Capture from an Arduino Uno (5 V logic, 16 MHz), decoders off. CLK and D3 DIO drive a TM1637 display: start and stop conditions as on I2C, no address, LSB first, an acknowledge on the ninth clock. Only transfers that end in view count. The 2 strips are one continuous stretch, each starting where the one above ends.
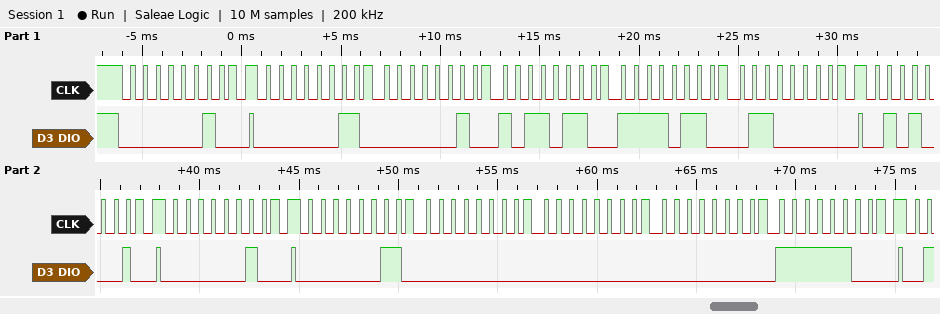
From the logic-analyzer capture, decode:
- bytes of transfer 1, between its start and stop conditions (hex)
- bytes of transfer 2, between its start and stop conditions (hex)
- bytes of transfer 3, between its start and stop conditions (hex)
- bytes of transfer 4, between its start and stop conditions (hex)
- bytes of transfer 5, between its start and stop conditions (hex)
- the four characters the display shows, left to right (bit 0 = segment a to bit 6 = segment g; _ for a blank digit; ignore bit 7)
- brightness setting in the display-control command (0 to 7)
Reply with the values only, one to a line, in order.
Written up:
40
C0 40 6D 6F 06
8A
40
C0 00 00 00 3F
___0
2
